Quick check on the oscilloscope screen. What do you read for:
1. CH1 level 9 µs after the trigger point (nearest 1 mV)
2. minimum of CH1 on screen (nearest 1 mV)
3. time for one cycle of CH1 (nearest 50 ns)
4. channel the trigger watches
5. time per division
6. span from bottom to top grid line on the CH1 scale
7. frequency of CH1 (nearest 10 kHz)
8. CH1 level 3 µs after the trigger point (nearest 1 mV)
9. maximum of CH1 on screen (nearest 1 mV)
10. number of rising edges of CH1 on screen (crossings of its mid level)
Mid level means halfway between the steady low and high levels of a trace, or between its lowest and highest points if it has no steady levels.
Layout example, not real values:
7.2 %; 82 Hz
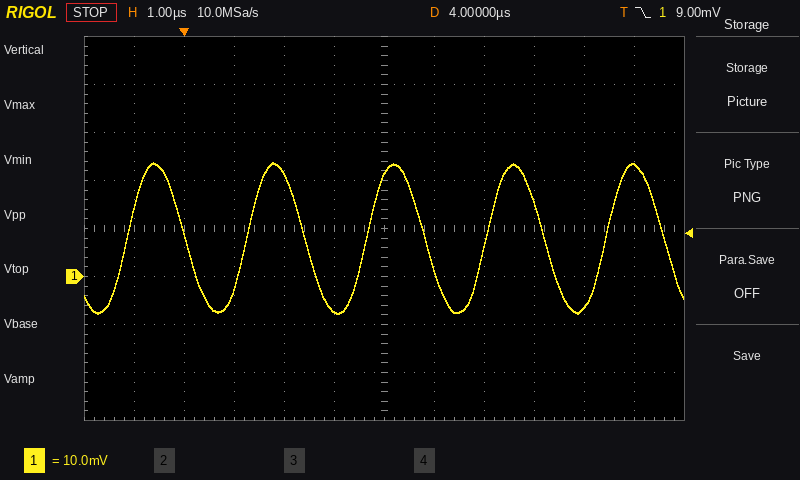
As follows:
23 mV; -8 mV; 2.40 µs; CH1; 1 µs; 80 mV; 420 kHz; -7 mV; 24 mV; 5
